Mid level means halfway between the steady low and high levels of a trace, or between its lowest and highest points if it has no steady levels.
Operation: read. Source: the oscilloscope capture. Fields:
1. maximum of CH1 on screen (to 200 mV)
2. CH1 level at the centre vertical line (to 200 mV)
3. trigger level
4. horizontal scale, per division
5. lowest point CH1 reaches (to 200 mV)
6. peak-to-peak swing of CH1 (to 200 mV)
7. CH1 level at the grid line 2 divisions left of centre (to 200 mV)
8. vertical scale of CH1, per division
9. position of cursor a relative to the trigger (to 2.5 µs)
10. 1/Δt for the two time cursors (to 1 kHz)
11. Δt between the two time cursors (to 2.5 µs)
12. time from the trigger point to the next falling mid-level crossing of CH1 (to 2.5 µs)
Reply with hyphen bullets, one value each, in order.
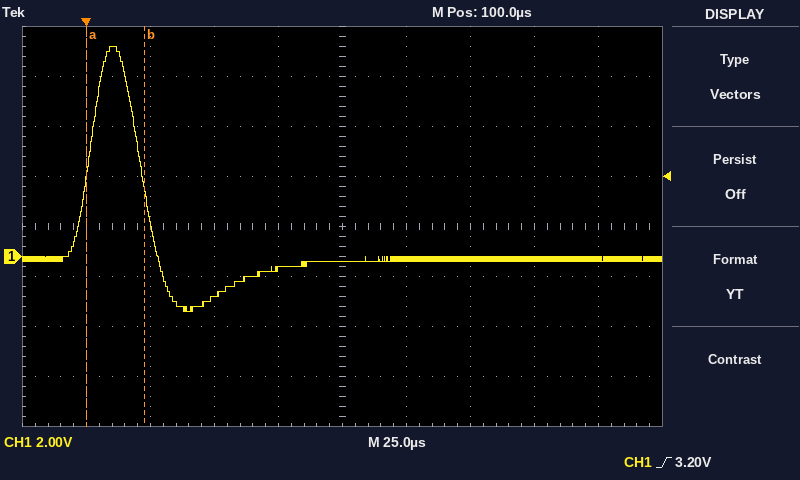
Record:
- 8.4 V
- -200 mV
- 3.20 V
- 25 µs
- -2.2 V
- 10.6 V
- -1.6 V
- 2 V
- 0.0 µs
- 44 kHz
- 22.5 µs
- 22.5 µs
